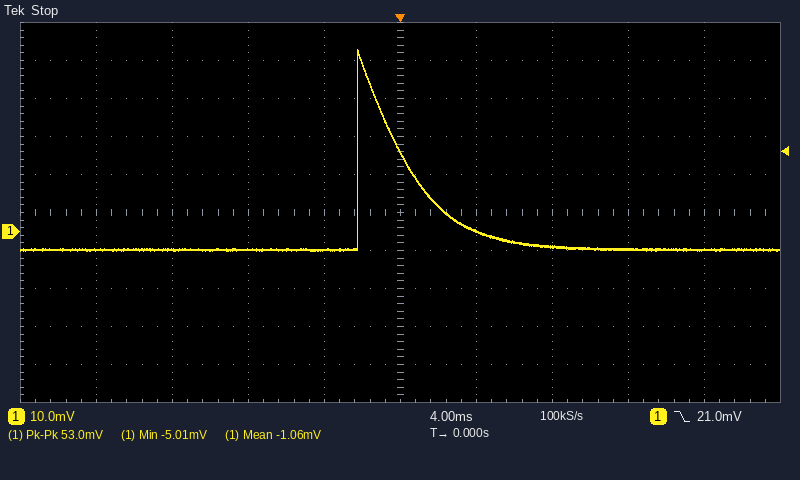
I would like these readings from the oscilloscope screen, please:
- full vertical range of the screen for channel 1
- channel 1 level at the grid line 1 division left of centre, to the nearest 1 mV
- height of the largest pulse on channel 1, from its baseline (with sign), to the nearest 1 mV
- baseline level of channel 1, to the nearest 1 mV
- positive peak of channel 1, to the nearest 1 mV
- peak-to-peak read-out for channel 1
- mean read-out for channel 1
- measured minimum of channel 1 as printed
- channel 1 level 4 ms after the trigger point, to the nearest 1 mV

100 mV
-5 mV
+53 mV
-5 mV
48 mV
53.0 mV
-1.06 mV
-5.01 mV
0 mV
